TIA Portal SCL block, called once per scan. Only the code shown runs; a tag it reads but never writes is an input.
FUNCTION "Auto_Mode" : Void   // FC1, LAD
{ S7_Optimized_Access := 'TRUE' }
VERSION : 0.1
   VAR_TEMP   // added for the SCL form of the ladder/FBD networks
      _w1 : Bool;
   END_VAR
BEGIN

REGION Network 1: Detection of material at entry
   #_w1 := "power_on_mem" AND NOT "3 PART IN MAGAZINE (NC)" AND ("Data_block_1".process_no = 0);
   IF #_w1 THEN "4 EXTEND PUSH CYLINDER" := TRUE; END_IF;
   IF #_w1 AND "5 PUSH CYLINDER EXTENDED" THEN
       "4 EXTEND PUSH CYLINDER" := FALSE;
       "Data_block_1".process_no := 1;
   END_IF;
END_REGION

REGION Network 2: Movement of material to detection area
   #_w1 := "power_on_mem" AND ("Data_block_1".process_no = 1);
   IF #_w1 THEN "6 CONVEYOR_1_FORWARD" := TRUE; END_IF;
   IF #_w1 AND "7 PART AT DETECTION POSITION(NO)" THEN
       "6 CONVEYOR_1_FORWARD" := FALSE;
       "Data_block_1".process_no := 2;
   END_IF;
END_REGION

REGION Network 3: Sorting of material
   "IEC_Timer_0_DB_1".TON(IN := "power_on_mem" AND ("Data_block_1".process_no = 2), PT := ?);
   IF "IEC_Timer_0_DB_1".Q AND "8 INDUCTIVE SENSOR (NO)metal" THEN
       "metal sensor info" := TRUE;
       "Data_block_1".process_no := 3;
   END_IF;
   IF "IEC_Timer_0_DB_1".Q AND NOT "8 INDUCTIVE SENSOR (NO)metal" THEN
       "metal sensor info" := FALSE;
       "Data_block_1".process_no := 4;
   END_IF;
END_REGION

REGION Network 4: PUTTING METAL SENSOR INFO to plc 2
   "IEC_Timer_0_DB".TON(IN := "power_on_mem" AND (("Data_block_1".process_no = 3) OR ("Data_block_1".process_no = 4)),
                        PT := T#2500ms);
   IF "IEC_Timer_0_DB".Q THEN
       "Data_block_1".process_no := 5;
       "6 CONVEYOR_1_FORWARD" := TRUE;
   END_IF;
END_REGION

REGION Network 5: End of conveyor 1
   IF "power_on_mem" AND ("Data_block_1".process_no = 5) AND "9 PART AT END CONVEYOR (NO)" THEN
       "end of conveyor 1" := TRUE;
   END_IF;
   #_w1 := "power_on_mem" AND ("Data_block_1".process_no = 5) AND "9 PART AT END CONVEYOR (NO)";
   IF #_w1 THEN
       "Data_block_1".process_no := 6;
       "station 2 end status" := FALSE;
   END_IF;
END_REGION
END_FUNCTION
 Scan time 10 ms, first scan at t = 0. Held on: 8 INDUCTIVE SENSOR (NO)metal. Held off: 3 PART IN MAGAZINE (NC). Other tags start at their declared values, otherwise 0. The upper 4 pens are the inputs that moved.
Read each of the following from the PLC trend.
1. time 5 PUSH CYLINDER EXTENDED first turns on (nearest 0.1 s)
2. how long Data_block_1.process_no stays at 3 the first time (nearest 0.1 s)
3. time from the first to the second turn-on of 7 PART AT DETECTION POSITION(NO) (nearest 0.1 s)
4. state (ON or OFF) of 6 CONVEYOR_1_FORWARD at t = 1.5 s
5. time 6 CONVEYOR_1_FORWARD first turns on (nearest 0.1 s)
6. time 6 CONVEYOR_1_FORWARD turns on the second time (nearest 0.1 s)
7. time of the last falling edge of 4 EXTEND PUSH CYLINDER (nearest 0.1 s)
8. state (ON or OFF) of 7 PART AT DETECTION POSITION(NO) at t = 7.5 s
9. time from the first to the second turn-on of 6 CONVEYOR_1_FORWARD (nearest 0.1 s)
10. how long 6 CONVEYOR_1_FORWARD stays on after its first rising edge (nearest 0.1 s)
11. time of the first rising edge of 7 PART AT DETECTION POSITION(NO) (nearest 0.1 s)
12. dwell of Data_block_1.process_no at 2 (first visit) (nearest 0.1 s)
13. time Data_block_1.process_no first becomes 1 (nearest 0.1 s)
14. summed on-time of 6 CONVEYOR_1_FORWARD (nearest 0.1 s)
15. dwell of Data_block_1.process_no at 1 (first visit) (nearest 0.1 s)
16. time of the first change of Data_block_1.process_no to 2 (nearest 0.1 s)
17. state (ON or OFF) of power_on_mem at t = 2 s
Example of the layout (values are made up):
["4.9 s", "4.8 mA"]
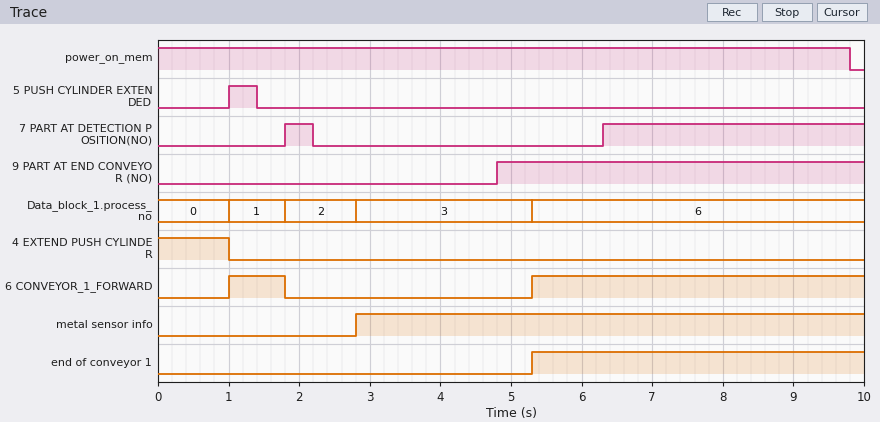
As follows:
["1.0 s", "2.5 s", "4.5 s", "ON", "1.0 s", "5.3 s", "1.0 s", "ON", "4.3 s", "0.8 s", "1.8 s", "1.0 s", "1.0 s", "5.5 s", "0.8 s", "1.8 s", "ON"]
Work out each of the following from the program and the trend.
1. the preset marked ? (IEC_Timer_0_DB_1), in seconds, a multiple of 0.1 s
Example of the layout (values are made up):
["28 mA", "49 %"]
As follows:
["1.0 s"]
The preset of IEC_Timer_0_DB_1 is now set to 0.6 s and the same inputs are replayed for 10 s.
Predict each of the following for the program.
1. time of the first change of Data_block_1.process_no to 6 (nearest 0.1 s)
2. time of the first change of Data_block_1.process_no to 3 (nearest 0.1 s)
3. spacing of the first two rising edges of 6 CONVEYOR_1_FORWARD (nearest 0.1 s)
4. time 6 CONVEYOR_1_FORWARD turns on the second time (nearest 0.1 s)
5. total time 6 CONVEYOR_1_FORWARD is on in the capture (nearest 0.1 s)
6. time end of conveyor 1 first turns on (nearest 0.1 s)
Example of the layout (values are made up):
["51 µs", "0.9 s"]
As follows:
["4.9 s", "2.4 s", "3.9 s", "4.9 s", "5.9 s", "4.9 s"]
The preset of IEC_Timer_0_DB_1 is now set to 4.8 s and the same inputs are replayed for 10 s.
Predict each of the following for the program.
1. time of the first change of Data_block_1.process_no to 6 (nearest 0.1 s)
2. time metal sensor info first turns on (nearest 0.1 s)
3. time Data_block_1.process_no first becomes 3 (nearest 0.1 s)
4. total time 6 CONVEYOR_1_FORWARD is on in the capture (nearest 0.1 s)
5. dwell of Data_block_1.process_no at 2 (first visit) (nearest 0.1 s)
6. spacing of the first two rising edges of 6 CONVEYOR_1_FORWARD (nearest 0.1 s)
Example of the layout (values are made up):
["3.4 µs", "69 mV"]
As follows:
["9.1 s", "6.6 s", "6.6 s", "1.7 s", "4.8 s", "8.1 s"]
